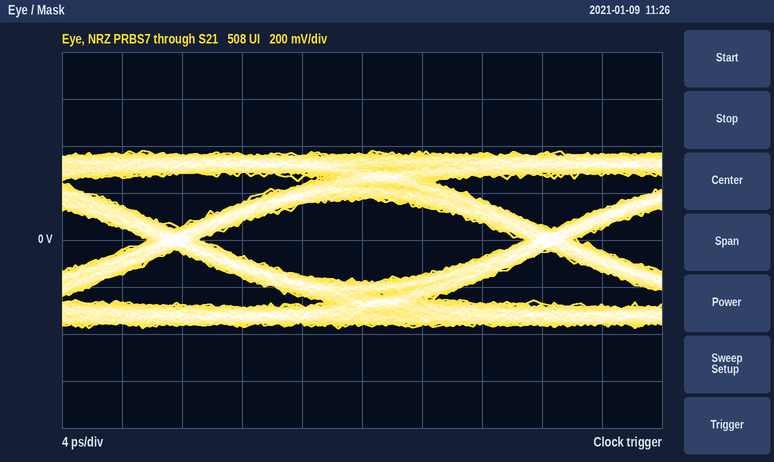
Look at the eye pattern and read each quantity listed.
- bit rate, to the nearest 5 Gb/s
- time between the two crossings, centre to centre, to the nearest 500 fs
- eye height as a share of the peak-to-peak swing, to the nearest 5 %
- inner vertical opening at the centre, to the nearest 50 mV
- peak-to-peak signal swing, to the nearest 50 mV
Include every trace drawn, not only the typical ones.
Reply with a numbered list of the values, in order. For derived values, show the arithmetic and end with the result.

1. 40 Gb/s
2. 25.0 ps
3. 350 mV / 750 mV ≈ 46.7 %, so 45 % to the nearest 5 %
4. 350 mV
5. 750 mV
